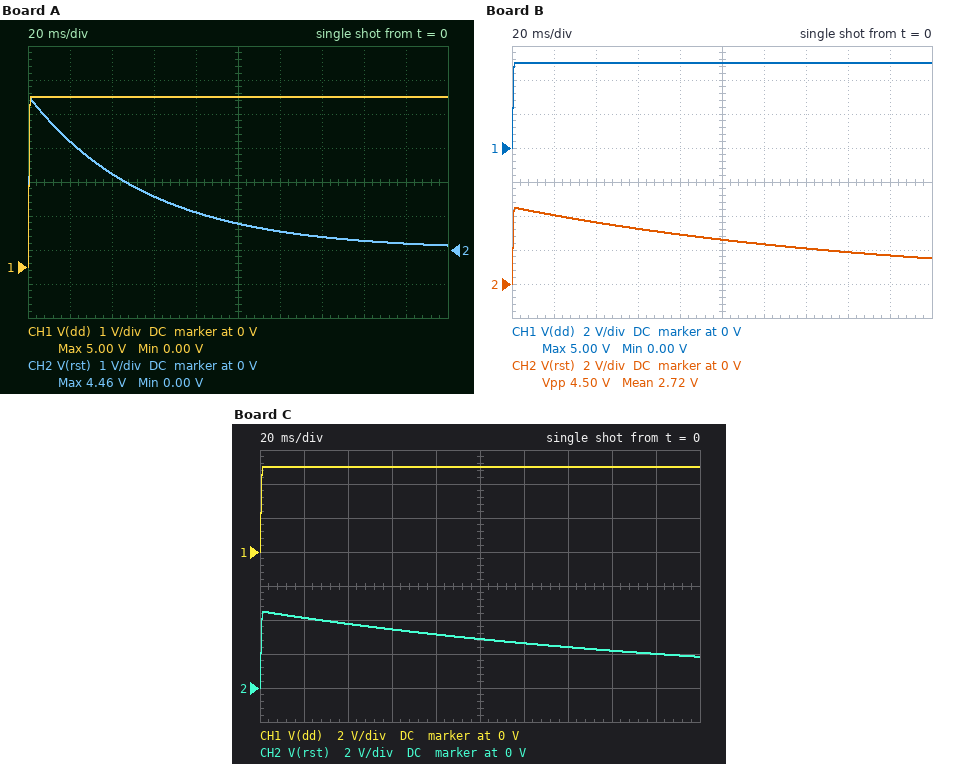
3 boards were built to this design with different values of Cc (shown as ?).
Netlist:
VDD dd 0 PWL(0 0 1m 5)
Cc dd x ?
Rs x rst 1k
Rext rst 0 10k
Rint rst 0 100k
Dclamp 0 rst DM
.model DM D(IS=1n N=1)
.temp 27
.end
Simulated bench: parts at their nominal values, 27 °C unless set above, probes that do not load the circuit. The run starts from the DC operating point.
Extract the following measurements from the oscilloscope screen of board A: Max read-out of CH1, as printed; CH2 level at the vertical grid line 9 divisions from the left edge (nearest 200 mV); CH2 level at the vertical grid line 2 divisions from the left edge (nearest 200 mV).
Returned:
5.00 V
200 mV
2.2 V
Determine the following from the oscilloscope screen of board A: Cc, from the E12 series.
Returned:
5.6 µF
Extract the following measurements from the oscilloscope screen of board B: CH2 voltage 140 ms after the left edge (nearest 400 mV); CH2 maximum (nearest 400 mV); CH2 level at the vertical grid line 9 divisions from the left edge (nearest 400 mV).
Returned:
2.0 V
4.4 V
1.6 V
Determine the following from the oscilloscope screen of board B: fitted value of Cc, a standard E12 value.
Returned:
18 µF
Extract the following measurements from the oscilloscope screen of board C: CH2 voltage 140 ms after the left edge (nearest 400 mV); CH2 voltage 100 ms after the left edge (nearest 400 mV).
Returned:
2.4 V
2.8 V
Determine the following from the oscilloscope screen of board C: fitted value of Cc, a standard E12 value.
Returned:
22 µF
